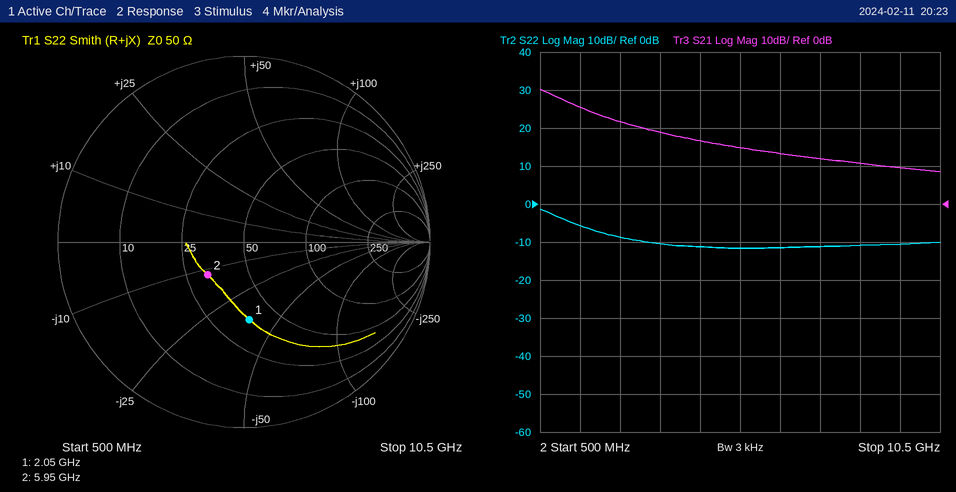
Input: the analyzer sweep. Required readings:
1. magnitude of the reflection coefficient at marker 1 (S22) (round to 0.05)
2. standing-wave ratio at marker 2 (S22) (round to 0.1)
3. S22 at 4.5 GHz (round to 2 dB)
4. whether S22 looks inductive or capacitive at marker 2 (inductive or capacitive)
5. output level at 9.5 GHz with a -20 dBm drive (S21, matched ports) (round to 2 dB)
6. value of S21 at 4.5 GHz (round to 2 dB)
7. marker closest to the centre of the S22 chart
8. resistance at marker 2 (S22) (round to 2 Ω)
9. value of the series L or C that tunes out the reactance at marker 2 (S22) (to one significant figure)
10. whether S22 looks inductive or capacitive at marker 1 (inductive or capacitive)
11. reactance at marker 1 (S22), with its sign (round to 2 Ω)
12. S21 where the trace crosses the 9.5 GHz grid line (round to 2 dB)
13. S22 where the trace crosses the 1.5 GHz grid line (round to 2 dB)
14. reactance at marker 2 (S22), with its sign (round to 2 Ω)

0.40
1.7
-12 dB
capacitive
-10 dBm
16 dB
marker 2
32 Ω
300 pH
capacitive
-38 Ω
10 dB
-6 dB
-12 Ω
